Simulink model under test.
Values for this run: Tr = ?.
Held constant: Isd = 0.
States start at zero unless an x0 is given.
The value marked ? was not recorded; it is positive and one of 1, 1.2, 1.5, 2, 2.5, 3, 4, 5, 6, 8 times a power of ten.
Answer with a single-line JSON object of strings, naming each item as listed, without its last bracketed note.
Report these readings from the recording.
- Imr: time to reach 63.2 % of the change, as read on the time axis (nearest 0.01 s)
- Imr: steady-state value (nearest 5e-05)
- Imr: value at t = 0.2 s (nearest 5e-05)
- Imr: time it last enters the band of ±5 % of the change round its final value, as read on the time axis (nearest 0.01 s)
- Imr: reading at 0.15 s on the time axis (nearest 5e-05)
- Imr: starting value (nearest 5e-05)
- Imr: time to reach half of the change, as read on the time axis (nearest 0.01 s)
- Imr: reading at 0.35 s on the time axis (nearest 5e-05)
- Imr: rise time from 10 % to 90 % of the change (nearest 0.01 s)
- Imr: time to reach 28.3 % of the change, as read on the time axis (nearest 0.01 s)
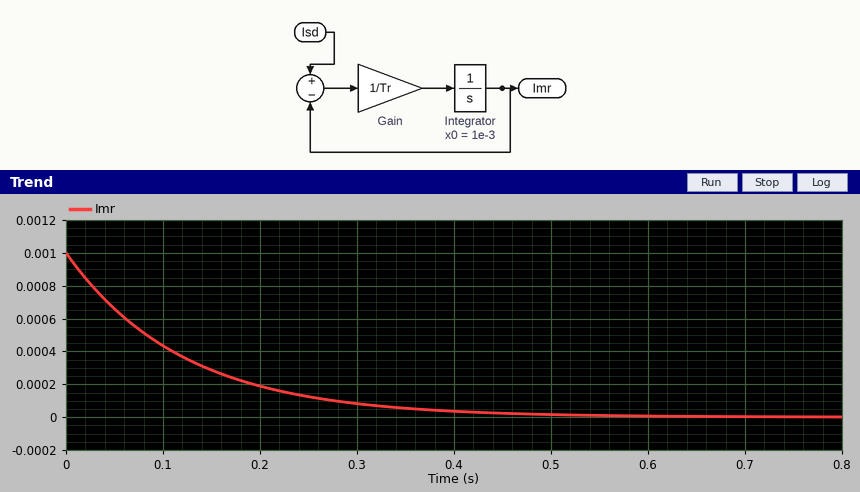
{"Imr: time to reach 63.2 % of the change, as read on the time axis": "0.12 s", "Imr: steady-state value": "0.00000", "Imr: value at t = 0.2 s": "0.00020", "Imr: time it last enters the band of ±5 % of the change round its final value, as read on the time axis": "0.36 s", "Imr: reading at 0.15 s on the time axis": "0.00030", "Imr: starting value": "0.00100", "Imr: time to reach half of the change, as read on the time axis": "0.08 s", "Imr: reading at 0.35 s on the time axis": "0.00005", "Imr: rise time from 10 % to 90 % of the change": "0.26 s", "Imr: time to reach 28.3 % of the change, as read on the time axis": "0.04 s"}
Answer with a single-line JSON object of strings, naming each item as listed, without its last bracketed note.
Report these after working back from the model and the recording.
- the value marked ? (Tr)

{"the value marked ?": "0.12"}
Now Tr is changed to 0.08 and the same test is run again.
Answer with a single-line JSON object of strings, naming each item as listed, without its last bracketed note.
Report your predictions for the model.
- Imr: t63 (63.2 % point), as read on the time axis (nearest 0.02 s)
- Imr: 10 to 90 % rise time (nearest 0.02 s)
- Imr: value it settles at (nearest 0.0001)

{"Imr: t63 (63.2 % point), as read on the time axis": "0.08 s", "Imr: 10 to 90 % rise time": "0.18 s", "Imr: value it settles at": "0.0000"}
